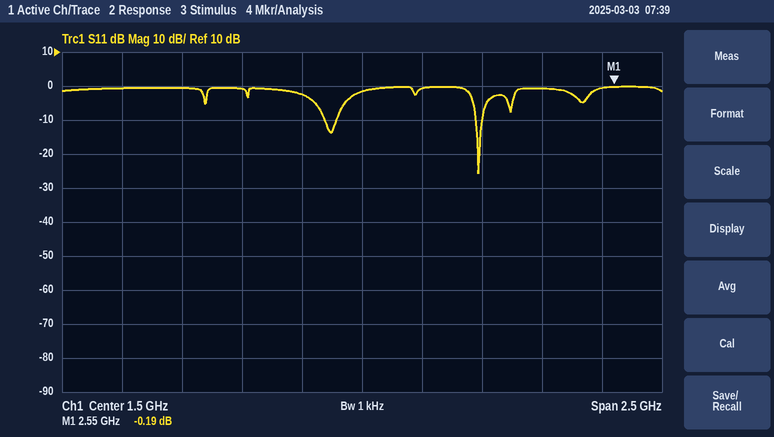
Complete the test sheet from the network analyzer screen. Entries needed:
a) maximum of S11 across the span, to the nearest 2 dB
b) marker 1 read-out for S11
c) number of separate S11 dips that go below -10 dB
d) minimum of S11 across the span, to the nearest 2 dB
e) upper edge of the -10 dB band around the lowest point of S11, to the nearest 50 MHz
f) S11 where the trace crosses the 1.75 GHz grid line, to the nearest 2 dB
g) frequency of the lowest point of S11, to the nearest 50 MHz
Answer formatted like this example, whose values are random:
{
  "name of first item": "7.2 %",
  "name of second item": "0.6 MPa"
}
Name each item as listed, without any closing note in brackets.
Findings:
{
  "maximum of S11 across the span, to the nearest 2 dB": "0 dB",
  "marker 1 read-out for S11": "-0.19 dB",
  "number of separate S11 dips that go below -10 dB": "2",
  "minimum of S11 across the span, to the nearest 2 dB": "-26 dB",
  "upper edge of the -10 dB band around the lowest point of S11, to the nearest 50 MHz": "2.00 GHz",
  "S11 where the trace crosses the 1.75 GHz grid line, to the nearest 2 dB": "0 dB",
  "frequency of the lowest point of S11, to the nearest 50 MHz": "2.00 GHz"
}
